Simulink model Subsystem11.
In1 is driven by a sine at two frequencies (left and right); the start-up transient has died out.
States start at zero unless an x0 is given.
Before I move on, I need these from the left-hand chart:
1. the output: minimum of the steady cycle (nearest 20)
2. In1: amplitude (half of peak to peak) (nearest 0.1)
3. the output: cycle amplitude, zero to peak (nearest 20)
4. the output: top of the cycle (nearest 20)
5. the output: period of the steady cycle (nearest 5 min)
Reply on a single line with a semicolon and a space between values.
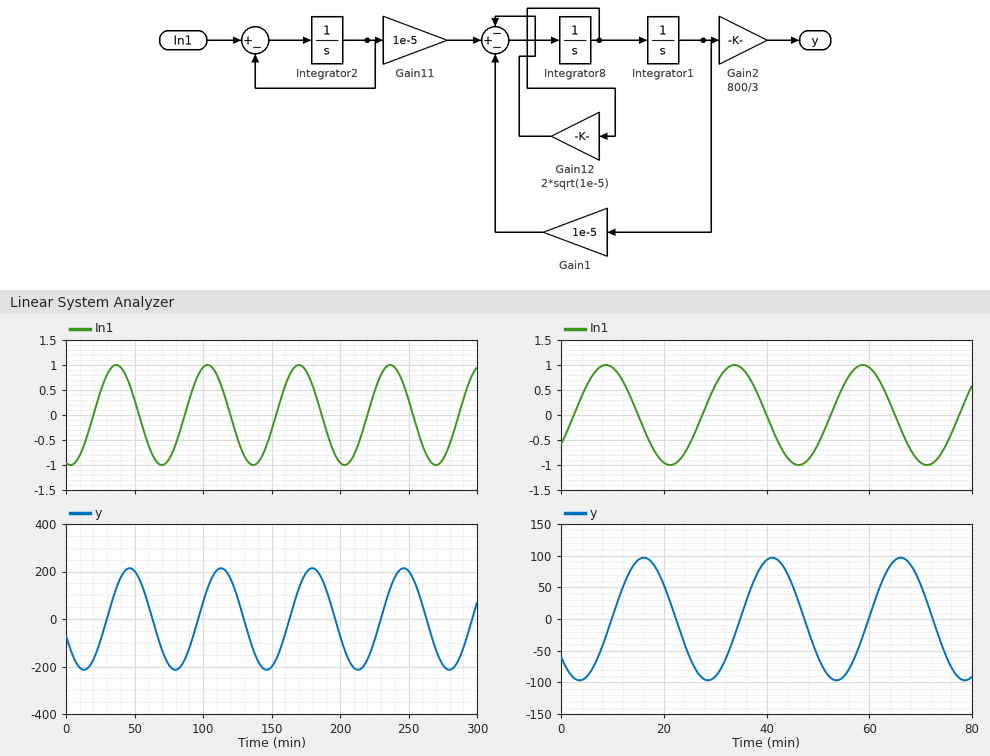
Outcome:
-220; 1.0; 220; 220; 65 min
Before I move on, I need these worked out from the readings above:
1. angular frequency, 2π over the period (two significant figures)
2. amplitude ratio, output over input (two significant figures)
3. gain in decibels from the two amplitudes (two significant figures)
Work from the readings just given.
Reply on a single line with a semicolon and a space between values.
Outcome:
0.097 rad/min; 220; 47 dB
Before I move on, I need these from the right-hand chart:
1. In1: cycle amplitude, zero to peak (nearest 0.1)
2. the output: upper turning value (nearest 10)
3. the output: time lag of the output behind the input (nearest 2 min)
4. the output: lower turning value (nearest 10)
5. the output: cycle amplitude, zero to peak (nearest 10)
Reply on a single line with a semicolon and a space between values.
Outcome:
1.0; 100; 8 min; -100; 100
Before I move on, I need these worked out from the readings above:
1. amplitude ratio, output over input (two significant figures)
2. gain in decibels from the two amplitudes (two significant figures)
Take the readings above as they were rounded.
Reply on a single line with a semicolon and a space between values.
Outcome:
100; 40 dB
